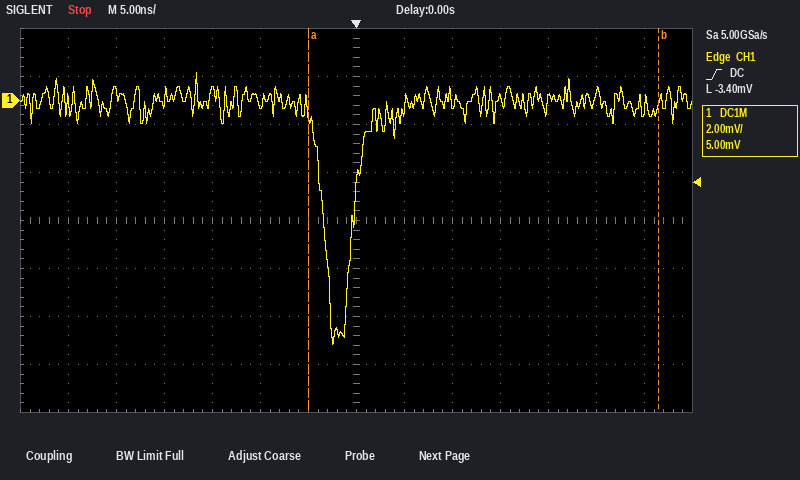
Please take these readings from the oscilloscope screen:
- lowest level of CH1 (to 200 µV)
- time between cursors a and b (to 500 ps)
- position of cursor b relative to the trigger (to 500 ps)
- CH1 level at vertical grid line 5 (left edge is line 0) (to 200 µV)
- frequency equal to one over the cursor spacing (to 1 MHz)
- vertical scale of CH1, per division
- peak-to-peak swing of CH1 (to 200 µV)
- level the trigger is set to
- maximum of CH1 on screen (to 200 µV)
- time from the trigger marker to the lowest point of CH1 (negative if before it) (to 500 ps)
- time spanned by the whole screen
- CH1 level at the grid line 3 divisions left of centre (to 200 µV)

-10.2 mV
36.5 ns
+31.5 ns
-200 µV
27 MHz
2 mV
11.4 mV
-3.40 mV
1.2 mV
-2.5 ns
70 ns
400 µV
